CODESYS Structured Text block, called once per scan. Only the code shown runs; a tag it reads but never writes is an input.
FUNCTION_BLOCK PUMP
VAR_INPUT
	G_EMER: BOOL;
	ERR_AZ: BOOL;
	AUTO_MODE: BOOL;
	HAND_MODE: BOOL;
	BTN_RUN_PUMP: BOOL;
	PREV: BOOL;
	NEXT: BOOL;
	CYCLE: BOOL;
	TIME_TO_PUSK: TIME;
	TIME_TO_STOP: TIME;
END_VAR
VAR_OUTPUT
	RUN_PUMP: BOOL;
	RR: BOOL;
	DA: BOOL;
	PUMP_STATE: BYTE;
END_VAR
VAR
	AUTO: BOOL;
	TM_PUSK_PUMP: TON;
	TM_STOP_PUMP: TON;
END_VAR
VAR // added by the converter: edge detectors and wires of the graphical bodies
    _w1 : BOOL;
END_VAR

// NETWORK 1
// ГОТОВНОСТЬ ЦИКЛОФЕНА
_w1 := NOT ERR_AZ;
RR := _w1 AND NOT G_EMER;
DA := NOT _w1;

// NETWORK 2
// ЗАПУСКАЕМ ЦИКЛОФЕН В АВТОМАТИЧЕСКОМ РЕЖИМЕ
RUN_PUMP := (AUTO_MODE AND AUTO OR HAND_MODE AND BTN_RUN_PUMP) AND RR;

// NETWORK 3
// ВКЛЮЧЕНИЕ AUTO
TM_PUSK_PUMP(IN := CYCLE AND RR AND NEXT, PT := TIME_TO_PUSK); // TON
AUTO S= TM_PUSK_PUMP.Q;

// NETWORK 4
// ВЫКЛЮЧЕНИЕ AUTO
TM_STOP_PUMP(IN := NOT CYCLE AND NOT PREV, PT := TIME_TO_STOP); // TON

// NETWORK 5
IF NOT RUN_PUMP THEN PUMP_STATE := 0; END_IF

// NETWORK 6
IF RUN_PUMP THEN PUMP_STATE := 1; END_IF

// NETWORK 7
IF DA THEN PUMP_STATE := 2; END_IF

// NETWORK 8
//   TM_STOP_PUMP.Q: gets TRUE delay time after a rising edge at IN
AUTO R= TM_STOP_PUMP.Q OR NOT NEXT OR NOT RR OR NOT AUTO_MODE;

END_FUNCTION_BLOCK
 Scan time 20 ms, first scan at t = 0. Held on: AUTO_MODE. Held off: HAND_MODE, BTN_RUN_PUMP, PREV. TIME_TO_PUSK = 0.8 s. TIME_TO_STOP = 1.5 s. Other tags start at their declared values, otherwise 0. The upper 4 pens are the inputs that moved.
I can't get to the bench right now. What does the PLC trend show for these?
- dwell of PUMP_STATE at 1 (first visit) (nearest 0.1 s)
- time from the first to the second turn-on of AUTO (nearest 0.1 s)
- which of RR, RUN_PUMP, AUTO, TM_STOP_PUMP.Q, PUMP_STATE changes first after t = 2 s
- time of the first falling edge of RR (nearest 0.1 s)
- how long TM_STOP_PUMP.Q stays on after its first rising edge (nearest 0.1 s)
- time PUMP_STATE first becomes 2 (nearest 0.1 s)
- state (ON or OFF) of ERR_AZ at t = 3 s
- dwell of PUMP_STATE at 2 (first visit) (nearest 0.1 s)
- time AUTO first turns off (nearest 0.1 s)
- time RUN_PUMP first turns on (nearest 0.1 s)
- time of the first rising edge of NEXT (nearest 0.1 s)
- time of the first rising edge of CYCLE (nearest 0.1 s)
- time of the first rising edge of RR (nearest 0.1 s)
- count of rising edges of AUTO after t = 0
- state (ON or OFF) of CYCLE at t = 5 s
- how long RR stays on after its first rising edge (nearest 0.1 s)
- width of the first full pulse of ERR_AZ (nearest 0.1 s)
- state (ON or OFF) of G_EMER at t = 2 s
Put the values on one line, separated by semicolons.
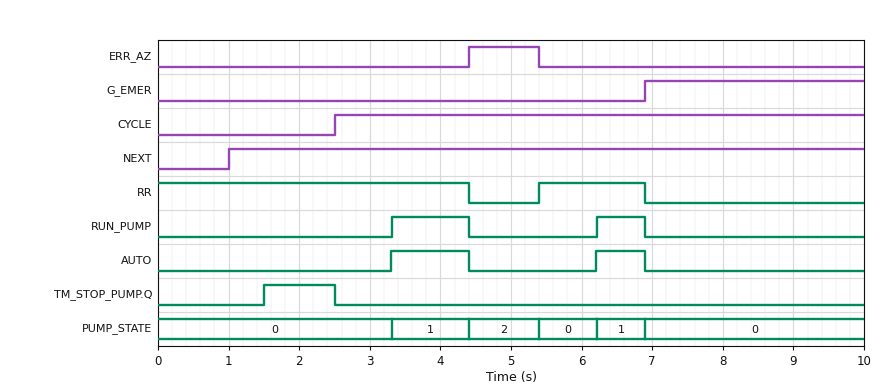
1.1 s; 2.9 s; TM_STOP_PUMP.Q; 4.4 s; 1.0 s; 4.4 s; OFF; 1.0 s; 4.4 s; 3.3 s; 1.0 s; 2.5 s; 5.4 s; 2; ON; 1.5 s; 1.0 s; OFF
